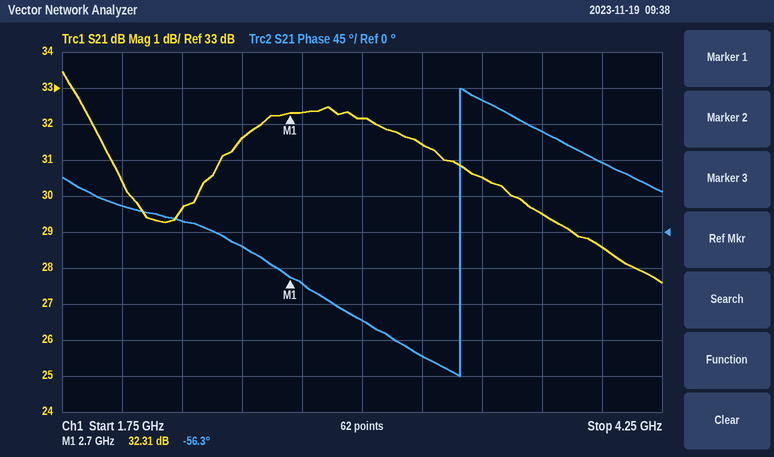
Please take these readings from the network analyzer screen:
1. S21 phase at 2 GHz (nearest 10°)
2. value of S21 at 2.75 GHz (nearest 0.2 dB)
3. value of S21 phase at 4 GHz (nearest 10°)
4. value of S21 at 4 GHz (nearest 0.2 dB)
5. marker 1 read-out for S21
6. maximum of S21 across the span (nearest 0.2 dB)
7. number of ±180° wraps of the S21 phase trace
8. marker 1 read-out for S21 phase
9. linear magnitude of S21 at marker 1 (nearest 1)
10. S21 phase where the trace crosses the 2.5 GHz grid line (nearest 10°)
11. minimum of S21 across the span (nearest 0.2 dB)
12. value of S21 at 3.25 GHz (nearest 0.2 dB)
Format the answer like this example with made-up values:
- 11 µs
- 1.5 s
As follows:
- 30°
- 32.4 dB
- 90°
- 28.6 dB
- 32.31 dB
- 33.4 dB
- 1
- -56.3°
- 41
- -20°
- 27.6 dB
- 31.4 dB
